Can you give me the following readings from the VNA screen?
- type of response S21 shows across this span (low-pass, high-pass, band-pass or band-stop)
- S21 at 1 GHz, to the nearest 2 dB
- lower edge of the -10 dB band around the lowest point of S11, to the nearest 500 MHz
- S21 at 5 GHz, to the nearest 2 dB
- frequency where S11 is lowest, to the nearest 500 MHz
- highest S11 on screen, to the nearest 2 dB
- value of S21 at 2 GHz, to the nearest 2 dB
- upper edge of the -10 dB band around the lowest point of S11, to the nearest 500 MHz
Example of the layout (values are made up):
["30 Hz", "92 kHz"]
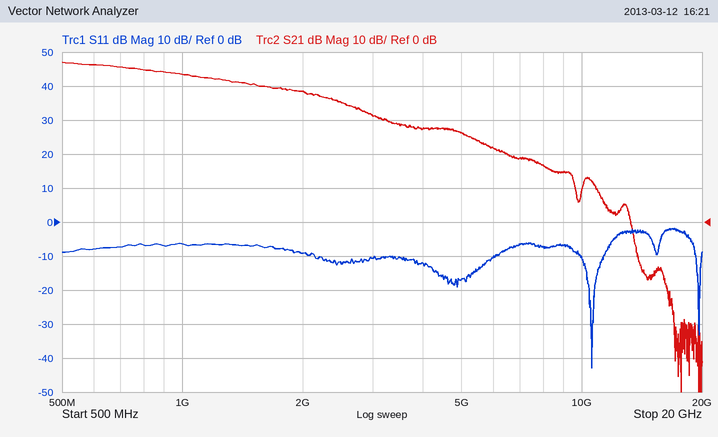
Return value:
["low-pass", "44 dB", "10.0 GHz", "26 dB", "10.5 GHz", "-2 dB", "38 dB", "11.5 GHz"]
